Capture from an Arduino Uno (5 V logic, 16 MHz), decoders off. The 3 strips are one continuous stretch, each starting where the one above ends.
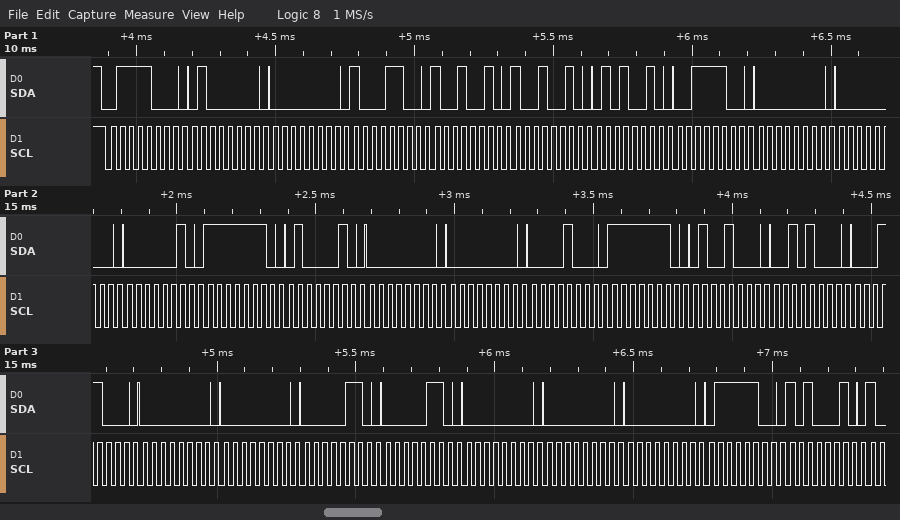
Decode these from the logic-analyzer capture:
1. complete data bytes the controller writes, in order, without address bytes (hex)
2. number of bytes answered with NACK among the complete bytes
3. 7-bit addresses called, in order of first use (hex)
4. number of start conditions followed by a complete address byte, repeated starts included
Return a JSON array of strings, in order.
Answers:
["40 00 8C 92 92 52 3C 00 00 02 FE 42 00 00 08 FE 48 28 18 00 00 06 06 00 00 00 7C A2", "0", "0x3C", "1"]
